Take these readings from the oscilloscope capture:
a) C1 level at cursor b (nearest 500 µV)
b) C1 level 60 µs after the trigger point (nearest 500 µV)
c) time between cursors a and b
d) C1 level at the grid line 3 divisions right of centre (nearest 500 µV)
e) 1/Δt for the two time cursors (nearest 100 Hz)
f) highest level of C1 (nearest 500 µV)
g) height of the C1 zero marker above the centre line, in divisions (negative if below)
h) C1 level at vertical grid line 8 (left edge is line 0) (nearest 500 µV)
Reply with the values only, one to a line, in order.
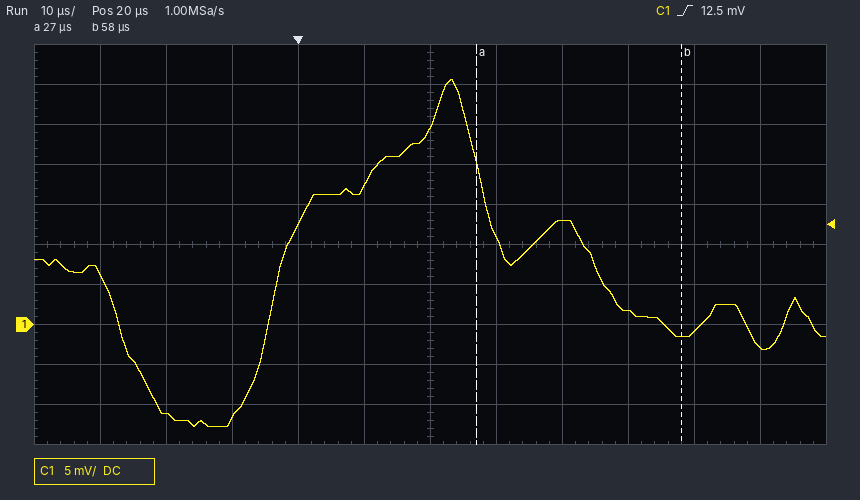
-1.5 mV
-1.0 mV
31 µs
1.5 mV
32.3 kHz
30.5 mV
-2.0 div
13.0 mV
